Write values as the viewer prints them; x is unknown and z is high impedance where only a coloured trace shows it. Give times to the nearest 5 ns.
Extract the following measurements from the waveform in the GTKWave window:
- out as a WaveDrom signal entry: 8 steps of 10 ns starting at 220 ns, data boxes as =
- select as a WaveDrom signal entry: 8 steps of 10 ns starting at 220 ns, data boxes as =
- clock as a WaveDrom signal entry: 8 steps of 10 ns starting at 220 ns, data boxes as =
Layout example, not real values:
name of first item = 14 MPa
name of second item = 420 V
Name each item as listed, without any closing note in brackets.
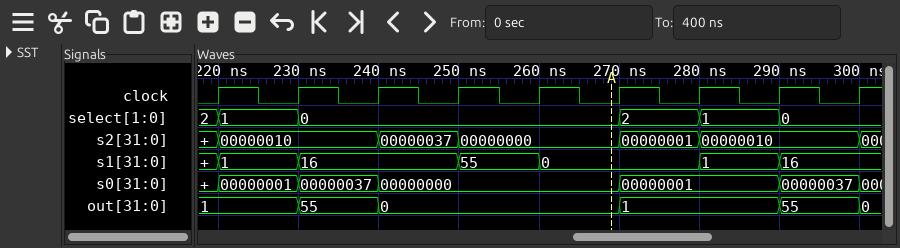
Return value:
out as a WaveDrom signal entry: 8 steps of 10 ns starting at 220 ns, data boxes as = = {name: 'out', wave: '===..=.=', data: '1 55 0 1 55'}
select as a WaveDrom signal entry: 8 steps of 10 ns starting at 220 ns, data boxes as = = {name: 'select', wave: '==...===', data: '1 0 2 1 0'}
clock as a WaveDrom signal entry: 8 steps of 10 ns starting at 220 ns, data boxes as = = {name: 'clock', wave: 'p.......'}
